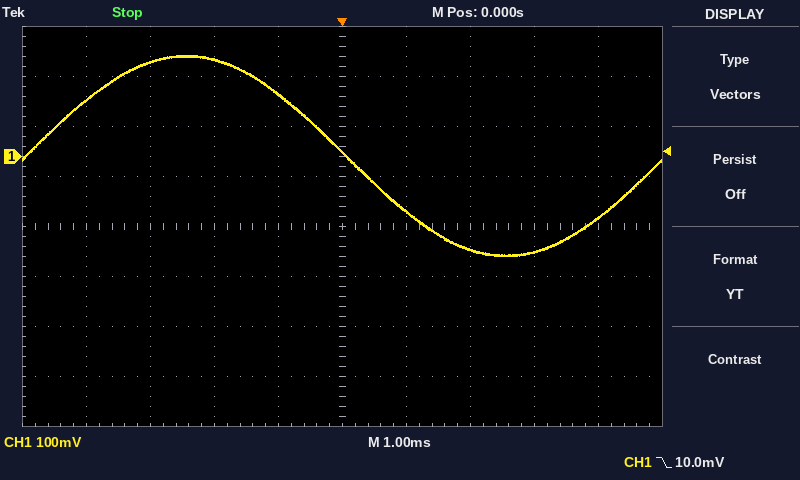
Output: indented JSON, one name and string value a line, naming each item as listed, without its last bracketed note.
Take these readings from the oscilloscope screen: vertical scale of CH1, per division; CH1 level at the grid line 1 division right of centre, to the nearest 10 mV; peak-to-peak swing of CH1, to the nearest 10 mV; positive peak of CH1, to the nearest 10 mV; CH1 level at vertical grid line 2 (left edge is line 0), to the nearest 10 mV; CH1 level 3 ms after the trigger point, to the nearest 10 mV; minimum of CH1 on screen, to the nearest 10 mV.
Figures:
{
  "vertical scale of CH1, per division": "100 mV",
  "CH1 level at the grid line 1 division right of centre, to the nearest 10 mV": "-110 mV",
  "peak-to-peak swing of CH1, to the nearest 10 mV": "400 mV",
  "positive peak of CH1, to the nearest 10 mV": "200 mV",
  "CH1 level at vertical grid line 2 (left edge is line 0), to the nearest 10 mV": "190 mV",
  "CH1 level 3 ms after the trigger point, to the nearest 10 mV": "-190 mV",
  "minimum of CH1 on screen, to the nearest 10 mV": "-200 mV"
}
